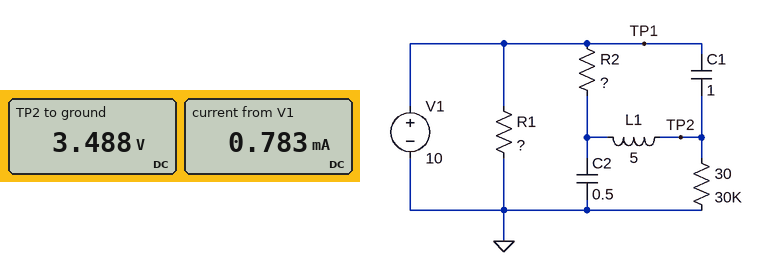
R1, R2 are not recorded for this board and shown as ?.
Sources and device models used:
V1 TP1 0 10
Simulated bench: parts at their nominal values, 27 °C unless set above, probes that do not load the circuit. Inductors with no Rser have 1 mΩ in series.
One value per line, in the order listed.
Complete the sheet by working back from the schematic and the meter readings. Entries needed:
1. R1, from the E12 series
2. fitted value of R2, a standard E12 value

15 kΩ
56 kΩ
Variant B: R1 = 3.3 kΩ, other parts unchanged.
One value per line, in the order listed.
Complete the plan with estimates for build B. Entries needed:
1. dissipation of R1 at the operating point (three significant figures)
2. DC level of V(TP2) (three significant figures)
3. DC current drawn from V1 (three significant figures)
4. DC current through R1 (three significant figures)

30.3 mW
3.49 V
3.15 mA
3.03 mA
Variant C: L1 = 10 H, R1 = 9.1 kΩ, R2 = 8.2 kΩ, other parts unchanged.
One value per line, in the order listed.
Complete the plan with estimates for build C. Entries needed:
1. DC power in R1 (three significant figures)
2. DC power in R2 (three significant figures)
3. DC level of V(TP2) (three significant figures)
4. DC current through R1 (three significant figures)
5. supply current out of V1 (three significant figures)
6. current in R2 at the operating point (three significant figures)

11.0 mW
562 µW
7.85 V
1.10 mA
1.36 mA
262 µA
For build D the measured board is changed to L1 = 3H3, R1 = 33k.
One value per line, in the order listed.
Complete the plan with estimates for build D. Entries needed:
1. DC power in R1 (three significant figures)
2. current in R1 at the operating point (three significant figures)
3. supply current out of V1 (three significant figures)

3.03 mW
303 µA
419 µA
